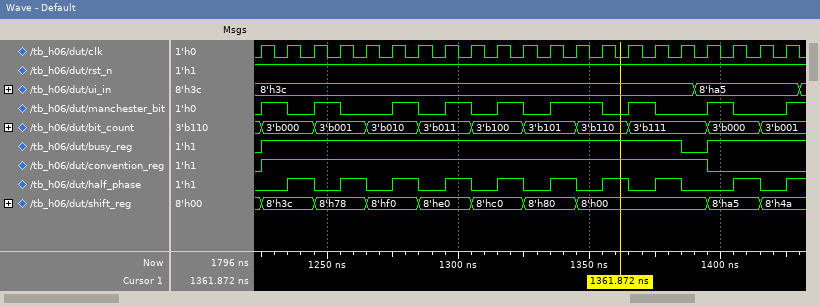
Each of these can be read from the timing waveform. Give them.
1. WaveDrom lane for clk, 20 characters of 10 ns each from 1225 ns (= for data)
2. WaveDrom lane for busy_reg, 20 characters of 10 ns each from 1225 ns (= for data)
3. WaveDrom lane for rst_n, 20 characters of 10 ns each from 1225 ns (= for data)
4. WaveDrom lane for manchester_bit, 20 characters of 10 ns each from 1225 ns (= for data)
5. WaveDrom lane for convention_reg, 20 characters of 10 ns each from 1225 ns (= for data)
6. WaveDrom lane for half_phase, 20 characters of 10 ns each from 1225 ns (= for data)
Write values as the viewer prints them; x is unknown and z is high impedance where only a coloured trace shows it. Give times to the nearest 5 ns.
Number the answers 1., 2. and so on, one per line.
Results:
1. {name: 'clk', wave: 'p...................'}
2. {name: 'busy_reg', wave: '1...............01..'}
3. {name: 'rst_n', wave: '1...................'}
4. {name: 'manchester_bit', wave: '1010.1010101.010.10.'}
5. {name: 'convention_reg', wave: '1................0..'}
6. {name: 'half_phase', wave: '01010101010101010.10'}
